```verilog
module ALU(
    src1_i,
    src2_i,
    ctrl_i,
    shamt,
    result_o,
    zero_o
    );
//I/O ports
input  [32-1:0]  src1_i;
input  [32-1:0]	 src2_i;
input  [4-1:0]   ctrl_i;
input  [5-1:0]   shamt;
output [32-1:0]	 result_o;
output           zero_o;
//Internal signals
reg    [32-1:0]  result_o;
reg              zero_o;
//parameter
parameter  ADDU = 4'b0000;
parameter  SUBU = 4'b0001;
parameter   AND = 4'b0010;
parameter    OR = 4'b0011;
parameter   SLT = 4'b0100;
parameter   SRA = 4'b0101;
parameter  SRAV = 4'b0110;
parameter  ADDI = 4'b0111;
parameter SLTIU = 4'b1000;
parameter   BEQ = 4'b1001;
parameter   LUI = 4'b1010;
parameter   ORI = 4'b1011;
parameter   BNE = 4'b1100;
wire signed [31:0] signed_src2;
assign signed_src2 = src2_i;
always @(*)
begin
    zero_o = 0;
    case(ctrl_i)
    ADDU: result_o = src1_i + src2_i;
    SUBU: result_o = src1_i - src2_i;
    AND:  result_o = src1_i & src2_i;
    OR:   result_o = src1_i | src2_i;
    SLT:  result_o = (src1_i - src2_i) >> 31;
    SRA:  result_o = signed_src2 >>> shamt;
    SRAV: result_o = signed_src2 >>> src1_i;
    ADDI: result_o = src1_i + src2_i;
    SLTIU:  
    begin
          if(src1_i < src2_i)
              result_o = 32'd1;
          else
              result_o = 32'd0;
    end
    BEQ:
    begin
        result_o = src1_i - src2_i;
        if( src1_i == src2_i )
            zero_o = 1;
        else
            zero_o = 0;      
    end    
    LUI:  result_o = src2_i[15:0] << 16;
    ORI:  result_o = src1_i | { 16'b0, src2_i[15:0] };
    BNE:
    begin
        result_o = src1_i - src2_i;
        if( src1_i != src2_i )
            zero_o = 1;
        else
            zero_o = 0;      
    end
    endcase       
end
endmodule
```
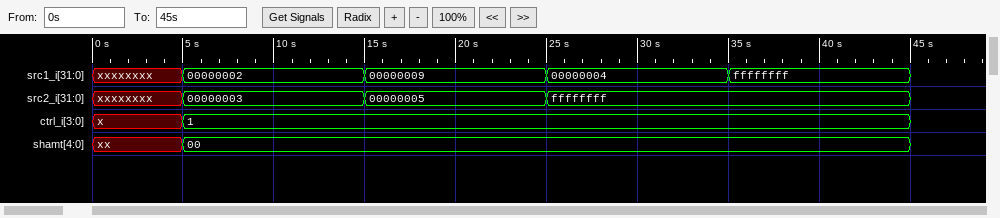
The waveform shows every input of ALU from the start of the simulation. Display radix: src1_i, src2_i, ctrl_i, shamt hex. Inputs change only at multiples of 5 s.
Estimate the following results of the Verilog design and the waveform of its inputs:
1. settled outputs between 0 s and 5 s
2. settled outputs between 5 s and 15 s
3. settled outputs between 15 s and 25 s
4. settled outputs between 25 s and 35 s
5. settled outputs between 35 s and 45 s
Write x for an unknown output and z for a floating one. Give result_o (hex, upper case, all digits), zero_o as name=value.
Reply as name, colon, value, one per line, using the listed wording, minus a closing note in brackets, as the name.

settled outputs between 0 s and 5 s: result_o=x, zero_o=x
settled outputs between 5 s and 15 s: result_o=FFFFFFFF, zero_o=0
settled outputs between 15 s and 25 s: result_o=00000004, zero_o=0
settled outputs between 25 s and 35 s: result_o=00000005, zero_o=0
settled outputs between 35 s and 45 s: result_o=00000000, zero_o=0
